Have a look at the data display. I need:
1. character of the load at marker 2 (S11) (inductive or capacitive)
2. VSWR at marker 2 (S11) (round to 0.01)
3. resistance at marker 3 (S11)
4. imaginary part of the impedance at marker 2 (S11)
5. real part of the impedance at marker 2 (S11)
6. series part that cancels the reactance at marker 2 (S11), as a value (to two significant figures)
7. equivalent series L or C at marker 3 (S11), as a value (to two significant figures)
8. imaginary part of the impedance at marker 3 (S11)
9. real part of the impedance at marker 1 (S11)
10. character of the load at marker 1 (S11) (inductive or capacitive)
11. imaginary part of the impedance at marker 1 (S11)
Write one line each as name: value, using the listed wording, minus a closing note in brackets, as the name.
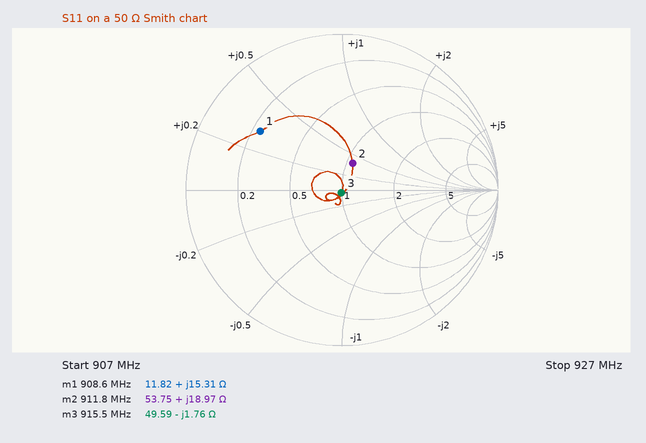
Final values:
character of the load at marker 2 (S11): inductive
VSWR at marker 2 (S11): 1.45
resistance at marker 3: 49.59 Ω
imaginary part of the impedance at marker 2: +18.97 Ω
real part of the impedance at marker 2: 53.75 Ω
series part that cancels the reactance at marker 2 (S11), as a value: 9.2 pF
equivalent series L or C at marker 3 (S11), as a value: 99 pF
imaginary part of the impedance at marker 3: -1.76 Ω
real part of the impedance at marker 1: 11.82 Ω
character of the load at marker 1 (S11): inductive
imaginary part of the impedance at marker 1: +15.31 Ω
